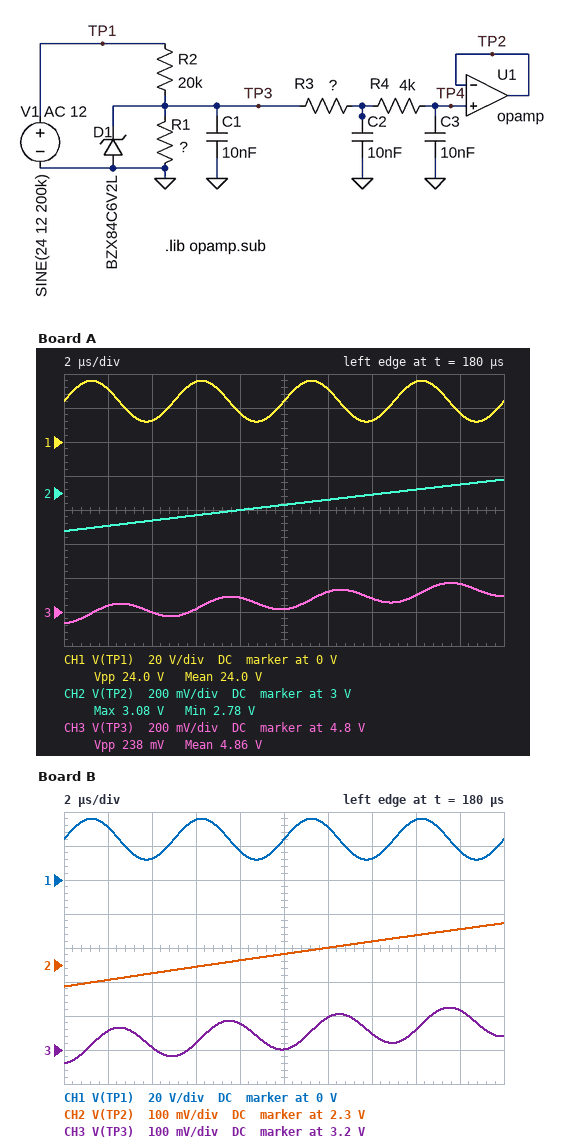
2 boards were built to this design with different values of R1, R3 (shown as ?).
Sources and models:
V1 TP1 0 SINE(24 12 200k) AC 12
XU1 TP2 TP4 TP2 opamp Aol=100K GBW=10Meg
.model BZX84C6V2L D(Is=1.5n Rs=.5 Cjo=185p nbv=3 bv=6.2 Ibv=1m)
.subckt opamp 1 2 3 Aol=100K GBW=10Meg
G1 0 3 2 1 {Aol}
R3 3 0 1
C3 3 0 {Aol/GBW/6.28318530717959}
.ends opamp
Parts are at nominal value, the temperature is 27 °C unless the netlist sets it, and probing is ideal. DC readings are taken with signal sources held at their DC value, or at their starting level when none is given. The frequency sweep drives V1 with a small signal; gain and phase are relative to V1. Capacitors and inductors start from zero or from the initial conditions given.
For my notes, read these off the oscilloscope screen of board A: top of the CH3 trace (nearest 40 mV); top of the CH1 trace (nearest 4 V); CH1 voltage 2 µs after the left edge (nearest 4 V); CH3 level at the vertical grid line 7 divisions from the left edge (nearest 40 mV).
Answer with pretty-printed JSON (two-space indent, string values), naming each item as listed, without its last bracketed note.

{
  "top of the CH3 trace": "4.96 V",
  "top of the CH1 trace": "36 V",
  "CH1 voltage 2 µs after the left edge": "32 V",
  "CH3 level at the vertical grid line 7 divisions from the left edge": "4.88 V"
}
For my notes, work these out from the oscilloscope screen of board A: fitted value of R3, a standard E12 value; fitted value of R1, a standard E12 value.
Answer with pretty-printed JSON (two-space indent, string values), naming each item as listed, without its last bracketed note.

{
  "fitted value of R3, a standard E12 value": "4.7 kΩ",
  "fitted value of R1, a standard E12 value": "8.2 kΩ"
}
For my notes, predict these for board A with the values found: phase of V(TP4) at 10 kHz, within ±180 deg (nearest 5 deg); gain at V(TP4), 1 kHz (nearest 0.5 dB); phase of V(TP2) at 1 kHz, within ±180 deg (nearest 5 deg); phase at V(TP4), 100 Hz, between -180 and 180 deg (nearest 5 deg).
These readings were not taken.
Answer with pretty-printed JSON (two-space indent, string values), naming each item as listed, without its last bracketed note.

{
  "phase of V(TP4) at 10 kHz, within ±180 deg": "-145 deg",
  "gain at V(TP4), 1 kHz": "-35.0 dB",
  "phase of V(TP2) at 1 kHz, within ±180 deg": "-45 deg",
  "phase at V(TP4), 100 Hz, between -180 and 180 deg": "-5 deg"
}
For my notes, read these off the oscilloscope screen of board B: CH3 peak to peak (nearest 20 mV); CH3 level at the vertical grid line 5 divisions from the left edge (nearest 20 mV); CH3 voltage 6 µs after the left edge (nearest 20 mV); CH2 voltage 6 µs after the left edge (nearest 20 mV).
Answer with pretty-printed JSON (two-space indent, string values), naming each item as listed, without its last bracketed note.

{
  "CH3 peak to peak": "160 mV",
  "CH3 level at the vertical grid line 5 divisions from the left edge": "3.20 V",
  "CH3 voltage 6 µs after the left edge": "3.22 V",
  "CH2 voltage 6 µs after the left edge": "2.30 V"
}
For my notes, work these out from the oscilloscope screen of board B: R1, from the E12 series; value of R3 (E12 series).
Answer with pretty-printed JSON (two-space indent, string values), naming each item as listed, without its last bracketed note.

{
  "R1, from the E12 series": "3.9 kΩ",
  "value of R3": "3.3 kΩ"
}
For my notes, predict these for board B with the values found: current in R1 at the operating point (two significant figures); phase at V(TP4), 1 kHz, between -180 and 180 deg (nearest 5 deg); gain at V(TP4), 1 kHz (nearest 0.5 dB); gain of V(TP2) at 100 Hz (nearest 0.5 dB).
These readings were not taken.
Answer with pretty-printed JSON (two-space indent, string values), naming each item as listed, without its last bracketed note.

{
  "current in R1 at the operating point": "1.0 mA",
  "phase at V(TP4), 1 kHz, between -180 and 180 deg": "-60 deg",
  "gain at V(TP4), 1 kHz": "-19.0 dB",
  "gain of V(TP2) at 100 Hz": "-16.0 dB"
}
